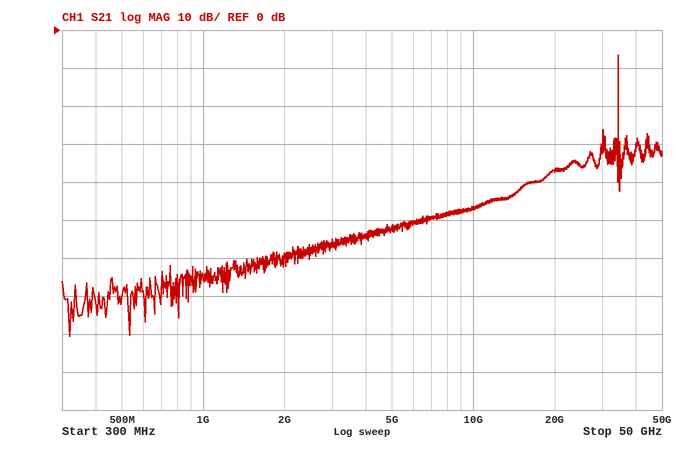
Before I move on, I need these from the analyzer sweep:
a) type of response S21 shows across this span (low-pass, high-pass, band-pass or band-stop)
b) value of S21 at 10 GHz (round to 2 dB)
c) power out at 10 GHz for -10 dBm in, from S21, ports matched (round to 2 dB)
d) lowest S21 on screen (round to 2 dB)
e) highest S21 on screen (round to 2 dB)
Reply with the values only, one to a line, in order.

band-pass
-46 dB
-56 dBm
-80 dB
-6 dB
